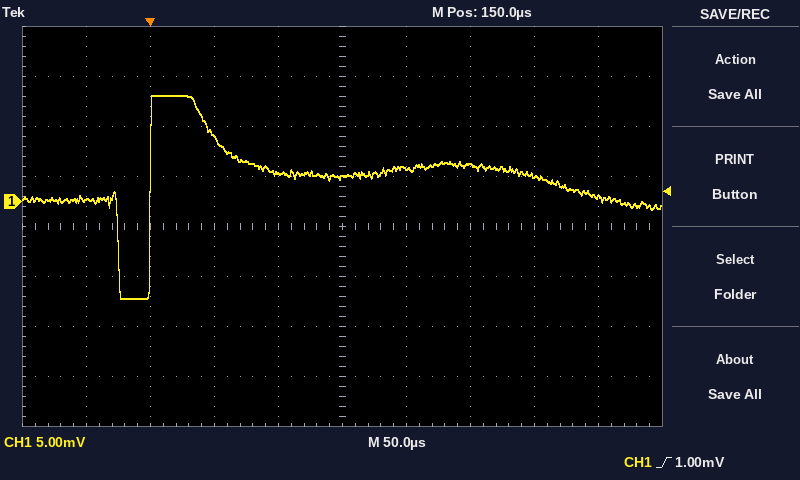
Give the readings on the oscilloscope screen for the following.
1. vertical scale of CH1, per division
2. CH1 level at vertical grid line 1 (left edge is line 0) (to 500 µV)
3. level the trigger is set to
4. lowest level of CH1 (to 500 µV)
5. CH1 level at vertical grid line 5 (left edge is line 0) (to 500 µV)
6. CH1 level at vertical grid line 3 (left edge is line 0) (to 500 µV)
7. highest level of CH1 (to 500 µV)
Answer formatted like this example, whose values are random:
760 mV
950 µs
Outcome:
5 mV
0.0 mV
1.00 mV
-9.5 mV
2.5 mV
6.5 mV
10.5 mV
